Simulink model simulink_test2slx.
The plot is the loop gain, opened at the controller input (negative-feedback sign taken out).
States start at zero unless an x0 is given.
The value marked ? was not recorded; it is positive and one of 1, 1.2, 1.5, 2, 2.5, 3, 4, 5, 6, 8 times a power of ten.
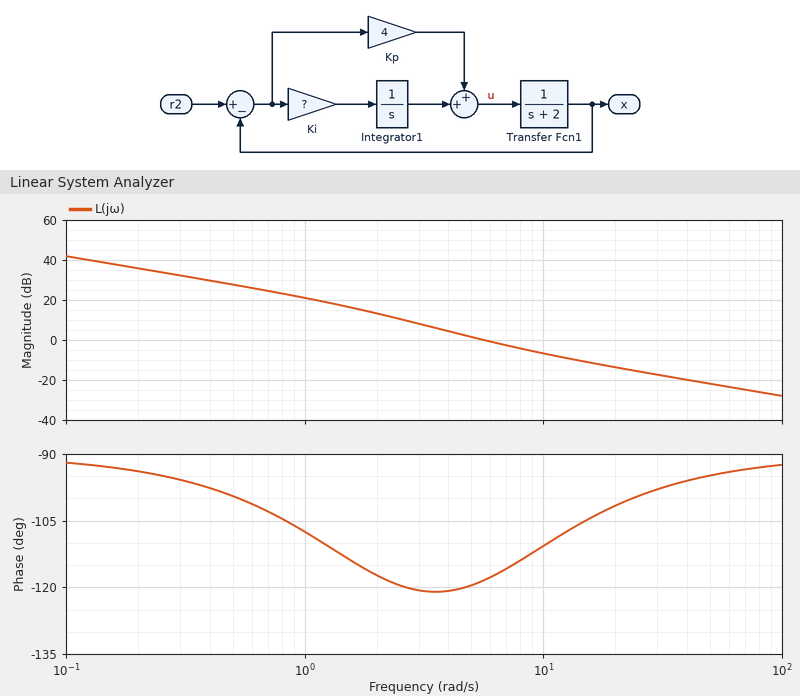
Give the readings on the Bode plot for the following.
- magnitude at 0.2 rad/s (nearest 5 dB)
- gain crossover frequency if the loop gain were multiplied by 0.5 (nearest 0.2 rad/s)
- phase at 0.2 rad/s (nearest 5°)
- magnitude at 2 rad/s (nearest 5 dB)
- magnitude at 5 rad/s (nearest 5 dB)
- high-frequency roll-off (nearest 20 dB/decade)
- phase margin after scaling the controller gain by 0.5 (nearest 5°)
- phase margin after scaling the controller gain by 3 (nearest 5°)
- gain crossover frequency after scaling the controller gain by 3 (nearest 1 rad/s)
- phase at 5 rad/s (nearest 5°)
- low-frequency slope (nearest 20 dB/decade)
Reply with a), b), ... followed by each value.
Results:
a) 35 dB
b) 3.6 rad/s
c) -95°
d) 15 dB
e) 0 dB
f) -20 dB/decade
g) 60°
h) 75°
i) 13 rad/s
j) -120°
k) -20 dB/decade
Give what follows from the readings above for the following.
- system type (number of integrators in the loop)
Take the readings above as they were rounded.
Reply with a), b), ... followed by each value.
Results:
a) 1
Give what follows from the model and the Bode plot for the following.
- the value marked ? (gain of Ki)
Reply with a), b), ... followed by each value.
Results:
a) 25
